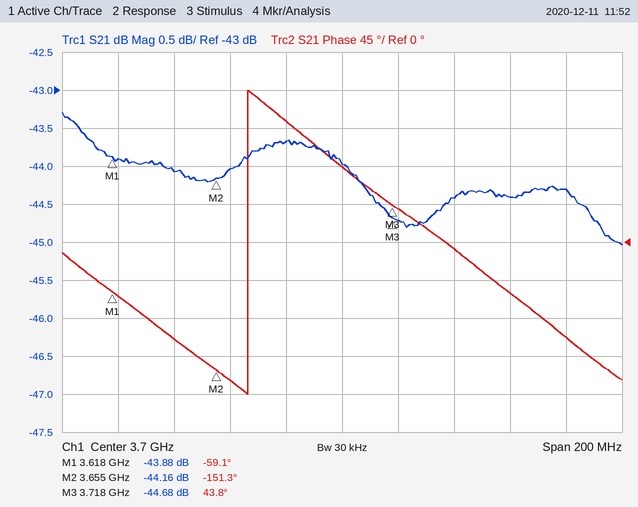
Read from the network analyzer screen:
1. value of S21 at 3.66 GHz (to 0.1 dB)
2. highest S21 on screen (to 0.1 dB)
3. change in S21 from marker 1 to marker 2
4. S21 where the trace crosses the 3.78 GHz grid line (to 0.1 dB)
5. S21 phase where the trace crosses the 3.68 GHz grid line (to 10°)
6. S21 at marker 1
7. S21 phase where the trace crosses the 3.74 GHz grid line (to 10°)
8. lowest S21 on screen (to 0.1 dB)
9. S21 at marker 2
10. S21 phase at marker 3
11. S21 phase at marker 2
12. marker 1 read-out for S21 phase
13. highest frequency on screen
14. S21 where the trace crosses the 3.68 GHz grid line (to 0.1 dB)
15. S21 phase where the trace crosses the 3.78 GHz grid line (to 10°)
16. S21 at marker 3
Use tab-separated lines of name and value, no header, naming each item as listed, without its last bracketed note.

value of S21 at 3.66 GHz	-44.0 dB
highest S21 on screen	-43.3 dB
change in S21 from marker 1 to marker 2	-0.28 dB
S21 where the trace crosses the 3.78 GHz grid line	-44.3 dB
S21 phase where the trace crosses the 3.68 GHz grid line	140°
S21 at marker 1	-43.88 dB
S21 phase where the trace crosses the 3.74 GHz grid line	-10°
lowest S21 on screen	-45.0 dB
S21 at marker 2	-44.16 dB
S21 phase at marker 3	43.8°
S21 phase at marker 2	-151.3°
marker 1 read-out for S21 phase	-59.1°
highest frequency on screen	3.8 GHz
S21 where the trace crosses the 3.68 GHz grid line	-43.7 dB
S21 phase where the trace crosses the 3.78 GHz grid line	-110°
S21 at marker 3	-44.68 dB
